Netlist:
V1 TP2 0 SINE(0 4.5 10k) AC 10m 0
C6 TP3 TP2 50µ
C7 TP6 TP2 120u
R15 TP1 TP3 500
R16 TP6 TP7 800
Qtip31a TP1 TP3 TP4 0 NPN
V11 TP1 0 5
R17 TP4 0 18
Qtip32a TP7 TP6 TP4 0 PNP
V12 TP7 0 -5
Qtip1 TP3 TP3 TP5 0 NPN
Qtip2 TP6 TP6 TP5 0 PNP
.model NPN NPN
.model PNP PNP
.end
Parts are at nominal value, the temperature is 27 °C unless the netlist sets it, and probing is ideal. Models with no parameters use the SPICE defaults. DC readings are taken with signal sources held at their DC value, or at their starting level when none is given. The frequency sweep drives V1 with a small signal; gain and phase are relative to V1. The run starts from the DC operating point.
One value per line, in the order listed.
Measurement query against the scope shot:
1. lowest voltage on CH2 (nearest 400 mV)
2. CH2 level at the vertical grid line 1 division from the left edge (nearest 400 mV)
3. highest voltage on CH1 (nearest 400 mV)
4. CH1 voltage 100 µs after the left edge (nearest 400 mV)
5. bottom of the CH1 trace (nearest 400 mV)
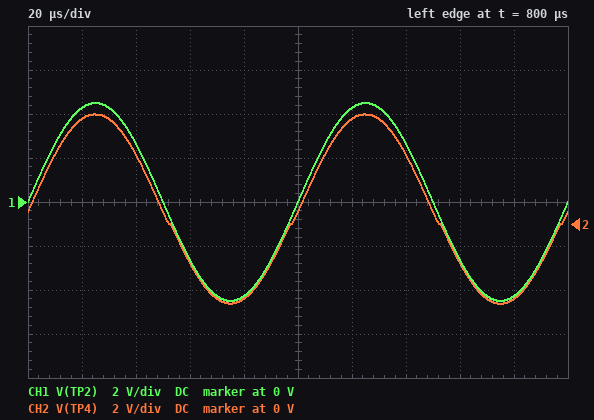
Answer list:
-3.6 V
4.8 V
4.4 V
0 V
-4.4 V
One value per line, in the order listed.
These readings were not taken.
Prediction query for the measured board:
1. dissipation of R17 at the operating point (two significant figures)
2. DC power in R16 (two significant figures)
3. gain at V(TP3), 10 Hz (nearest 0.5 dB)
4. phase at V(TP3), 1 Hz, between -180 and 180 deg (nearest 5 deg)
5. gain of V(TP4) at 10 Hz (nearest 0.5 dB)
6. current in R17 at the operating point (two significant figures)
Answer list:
34 mW
31 mW
-0.5 dB
75 deg
-1.0 dB
43 mA
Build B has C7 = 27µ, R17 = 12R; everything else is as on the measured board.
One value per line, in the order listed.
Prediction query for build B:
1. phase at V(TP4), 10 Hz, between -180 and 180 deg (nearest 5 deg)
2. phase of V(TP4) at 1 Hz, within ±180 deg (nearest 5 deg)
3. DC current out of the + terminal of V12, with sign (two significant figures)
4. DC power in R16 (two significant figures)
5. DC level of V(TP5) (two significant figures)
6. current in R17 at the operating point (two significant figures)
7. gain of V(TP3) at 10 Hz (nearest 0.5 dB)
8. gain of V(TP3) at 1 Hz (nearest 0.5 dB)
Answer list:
40 deg
85 deg
-6.8 mA
31 mW
780 mV
60 mA
-2.5 dB
-18.5 dB
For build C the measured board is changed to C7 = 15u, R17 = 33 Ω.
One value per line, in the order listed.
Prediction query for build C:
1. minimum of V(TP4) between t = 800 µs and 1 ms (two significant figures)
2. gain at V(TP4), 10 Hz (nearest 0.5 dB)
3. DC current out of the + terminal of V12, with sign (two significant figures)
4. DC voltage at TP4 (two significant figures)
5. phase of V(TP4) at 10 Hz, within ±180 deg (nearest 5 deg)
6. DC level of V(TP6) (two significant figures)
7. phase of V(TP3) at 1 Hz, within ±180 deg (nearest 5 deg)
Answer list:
-3.8 V
-2.5 dB
-7.8 mA
850 mV
40 deg
64 mV
85 deg
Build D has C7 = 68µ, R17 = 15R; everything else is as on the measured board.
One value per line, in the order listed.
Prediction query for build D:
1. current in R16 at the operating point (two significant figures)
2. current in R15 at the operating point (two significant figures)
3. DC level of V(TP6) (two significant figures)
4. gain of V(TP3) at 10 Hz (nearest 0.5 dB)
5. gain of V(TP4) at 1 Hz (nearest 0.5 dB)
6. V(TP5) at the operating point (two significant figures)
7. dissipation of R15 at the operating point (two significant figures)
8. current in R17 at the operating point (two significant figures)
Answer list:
6.2 mA
6.7 mA
-11 mV
-1.0 dB
-15.0 dB
810 mV
23 mW
50 mA
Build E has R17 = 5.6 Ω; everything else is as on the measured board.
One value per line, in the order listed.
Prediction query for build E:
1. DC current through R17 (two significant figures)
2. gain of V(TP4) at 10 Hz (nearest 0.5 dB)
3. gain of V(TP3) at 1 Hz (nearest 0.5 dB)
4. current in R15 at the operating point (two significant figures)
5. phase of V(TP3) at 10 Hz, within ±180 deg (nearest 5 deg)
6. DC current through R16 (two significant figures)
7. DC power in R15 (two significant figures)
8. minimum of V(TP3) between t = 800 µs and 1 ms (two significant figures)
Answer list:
100 mA
-1.5 dB
-13.5 dB
7.1 mA
25 deg
6.0 mA
25 mW
-3.1 V
